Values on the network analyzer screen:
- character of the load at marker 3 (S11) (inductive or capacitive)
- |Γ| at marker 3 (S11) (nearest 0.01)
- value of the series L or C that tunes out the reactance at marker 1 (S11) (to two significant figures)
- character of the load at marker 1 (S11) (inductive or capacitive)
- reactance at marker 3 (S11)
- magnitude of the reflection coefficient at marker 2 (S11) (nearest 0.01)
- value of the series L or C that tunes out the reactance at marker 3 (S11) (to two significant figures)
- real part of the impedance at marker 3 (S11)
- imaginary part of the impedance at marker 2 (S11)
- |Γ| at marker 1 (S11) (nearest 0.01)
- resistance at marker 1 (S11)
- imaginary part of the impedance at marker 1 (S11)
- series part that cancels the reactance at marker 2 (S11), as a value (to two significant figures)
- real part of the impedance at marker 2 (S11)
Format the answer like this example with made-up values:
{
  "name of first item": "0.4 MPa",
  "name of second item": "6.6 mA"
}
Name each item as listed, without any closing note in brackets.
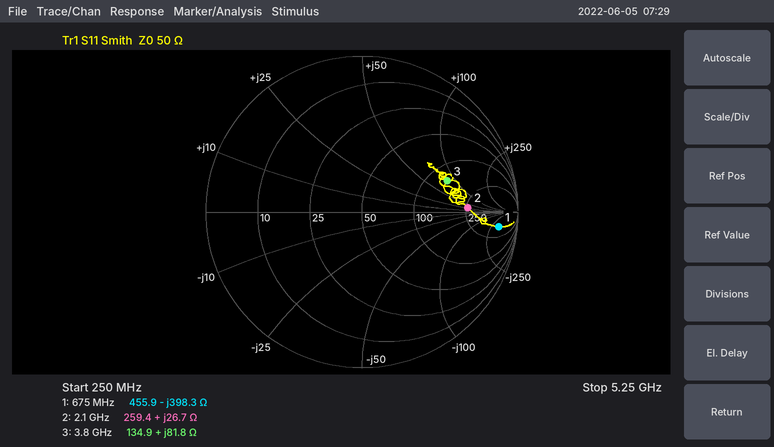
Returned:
{
  "character of the load at marker 3 (S11)": "inductive",
  "|Γ| at marker 3 (S11)": "0.58",
  "value of the series L or C that tunes out the reactance at marker 1 (S11)": "94 nH",
  "character of the load at marker 1 (S11)": "capacitive",
  "reactance at marker 3": "+81.8 Ω",
  "magnitude of the reflection coefficient at marker 2 (S11)": "0.68",
  "value of the series L or C that tunes out the reactance at marker 3 (S11)": "510 fF",
  "real part of the impedance at marker 3": "134.9 Ω",
  "imaginary part of the impedance at marker 2": "+26.7 Ω",
  "|Γ| at marker 1 (S11)": "0.88",
  "resistance at marker 1": "455.9 Ω",
  "imaginary part of the impedance at marker 1": "-398.3 Ω",
  "series part that cancels the reactance at marker 2 (S11), as a value": "2.8 pF",
  "real part of the impedance at marker 2": "259.4 Ω"
}
